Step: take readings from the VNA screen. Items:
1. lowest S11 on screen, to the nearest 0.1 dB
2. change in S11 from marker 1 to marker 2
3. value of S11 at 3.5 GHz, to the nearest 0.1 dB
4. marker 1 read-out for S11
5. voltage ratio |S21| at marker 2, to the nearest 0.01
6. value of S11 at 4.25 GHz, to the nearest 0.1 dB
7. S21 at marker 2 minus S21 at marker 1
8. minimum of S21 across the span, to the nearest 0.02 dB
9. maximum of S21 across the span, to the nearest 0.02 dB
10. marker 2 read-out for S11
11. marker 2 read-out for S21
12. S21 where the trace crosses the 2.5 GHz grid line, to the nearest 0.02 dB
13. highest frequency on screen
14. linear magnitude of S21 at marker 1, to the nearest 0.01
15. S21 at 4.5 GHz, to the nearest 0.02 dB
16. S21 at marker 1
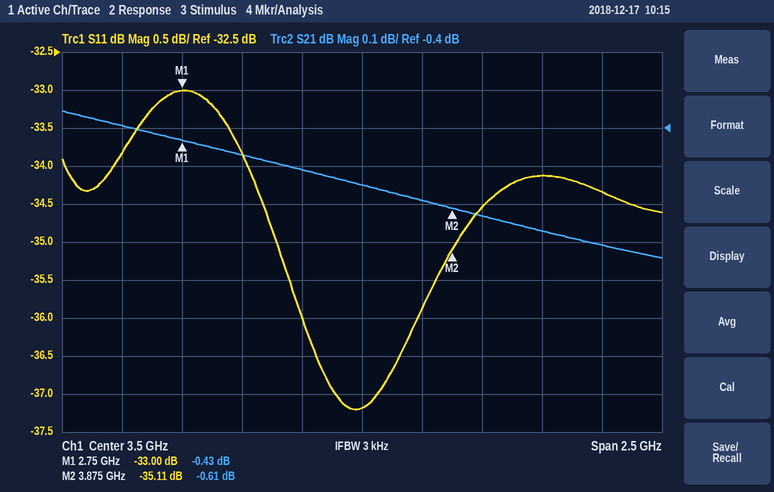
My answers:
-37.2 dB
-2.11 dB
-37.2 dB
-33.00 dB
0.93
-34.1 dB
-0.18 dB
-0.74 dB
-0.36 dB
-35.11 dB
-0.61 dB
-0.40 dB
4.75 GHz
0.95
-0.70 dB
-0.43 dB
